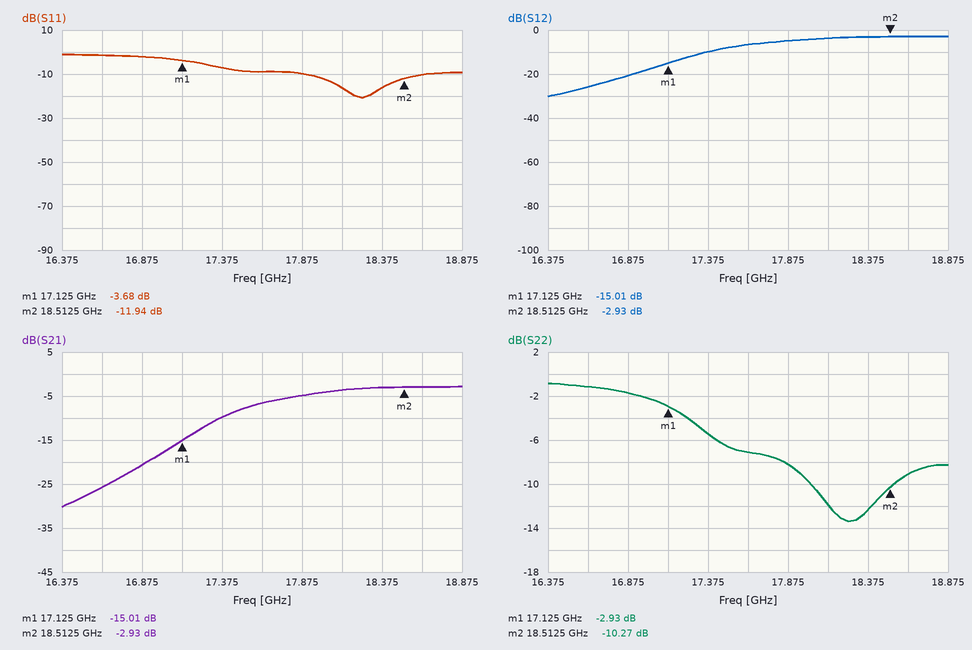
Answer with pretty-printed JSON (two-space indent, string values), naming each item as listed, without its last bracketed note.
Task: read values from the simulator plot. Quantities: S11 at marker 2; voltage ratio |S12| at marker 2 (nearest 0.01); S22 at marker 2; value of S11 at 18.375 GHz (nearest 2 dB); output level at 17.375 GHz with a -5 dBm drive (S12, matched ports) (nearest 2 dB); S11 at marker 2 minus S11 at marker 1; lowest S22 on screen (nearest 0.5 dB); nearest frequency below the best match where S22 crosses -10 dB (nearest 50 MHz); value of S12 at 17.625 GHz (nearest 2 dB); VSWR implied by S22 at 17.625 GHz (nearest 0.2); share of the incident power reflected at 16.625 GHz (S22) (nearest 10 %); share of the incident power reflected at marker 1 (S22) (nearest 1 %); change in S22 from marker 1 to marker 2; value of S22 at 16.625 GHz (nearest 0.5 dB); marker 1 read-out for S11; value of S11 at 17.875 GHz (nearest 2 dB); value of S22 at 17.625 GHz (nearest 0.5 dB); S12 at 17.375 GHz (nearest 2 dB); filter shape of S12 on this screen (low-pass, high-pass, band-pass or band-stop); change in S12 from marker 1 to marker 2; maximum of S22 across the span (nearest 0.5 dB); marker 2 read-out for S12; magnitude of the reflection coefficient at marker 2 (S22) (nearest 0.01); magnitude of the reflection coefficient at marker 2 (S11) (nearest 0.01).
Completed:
{
  "S11 at marker 2": "-11.94 dB",
  "voltage ratio |S12| at marker 2": "0.71",
  "S22 at marker 2": "-10.27 dB",
  "value of S11 at 18.375 GHz": "-16 dB",
  "output level at 17.375 GHz with a -5 dBm drive (S12, matched ports)": "-14 dBm",
  "S11 at marker 2 minus S11 at marker 1": "-8.26 dB",
  "lowest S22 on screen": "-13.5 dB",
  "nearest frequency below the best match where S22 crosses -10 dB": "18.00 GHz",
  "value of S12 at 17.625 GHz": "-6 dB",
  "VSWR implied by S22 at 17.625 GHz": "2.6",
  "share of the incident power reflected at 16.625 GHz (S22)": "80 %",
  "share of the incident power reflected at marker 1 (S22)": "51 %",
  "change in S22 from marker 1 to marker 2": "-7.34 dB",
  "value of S22 at 16.625 GHz": "-1.0 dB",
  "marker 1 read-out for S11": "-3.68 dB",
  "value of S11 at 17.875 GHz": "-10 dB",
  "value of S22 at 17.625 GHz": "-7.0 dB",
  "S12 at 17.375 GHz": "-10 dB",
  "filter shape of S12 on this screen": "high-pass",
  "change in S12 from marker 1 to marker 2": "12.08 dB",
  "maximum of S22 across the span": "-1.0 dB",
  "marker 2 read-out for S12": "-2.93 dB",
  "magnitude of the reflection coefficient at marker 2 (S22)": "0.31",
  "magnitude of the reflection coefficient at marker 2 (S11)": "0.25"
}
